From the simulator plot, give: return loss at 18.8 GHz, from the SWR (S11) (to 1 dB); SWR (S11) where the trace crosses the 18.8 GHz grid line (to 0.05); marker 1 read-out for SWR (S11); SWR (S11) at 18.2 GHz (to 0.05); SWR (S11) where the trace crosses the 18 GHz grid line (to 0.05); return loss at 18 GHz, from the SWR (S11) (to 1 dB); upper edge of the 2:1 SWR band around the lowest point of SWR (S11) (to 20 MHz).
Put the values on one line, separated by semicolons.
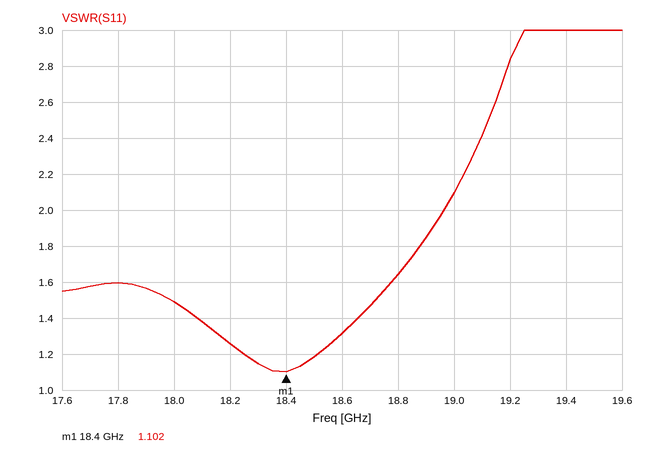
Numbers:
12 dB; 1.65; 1.102; 1.25; 1.50; 14 dB; 18.96 GHz
